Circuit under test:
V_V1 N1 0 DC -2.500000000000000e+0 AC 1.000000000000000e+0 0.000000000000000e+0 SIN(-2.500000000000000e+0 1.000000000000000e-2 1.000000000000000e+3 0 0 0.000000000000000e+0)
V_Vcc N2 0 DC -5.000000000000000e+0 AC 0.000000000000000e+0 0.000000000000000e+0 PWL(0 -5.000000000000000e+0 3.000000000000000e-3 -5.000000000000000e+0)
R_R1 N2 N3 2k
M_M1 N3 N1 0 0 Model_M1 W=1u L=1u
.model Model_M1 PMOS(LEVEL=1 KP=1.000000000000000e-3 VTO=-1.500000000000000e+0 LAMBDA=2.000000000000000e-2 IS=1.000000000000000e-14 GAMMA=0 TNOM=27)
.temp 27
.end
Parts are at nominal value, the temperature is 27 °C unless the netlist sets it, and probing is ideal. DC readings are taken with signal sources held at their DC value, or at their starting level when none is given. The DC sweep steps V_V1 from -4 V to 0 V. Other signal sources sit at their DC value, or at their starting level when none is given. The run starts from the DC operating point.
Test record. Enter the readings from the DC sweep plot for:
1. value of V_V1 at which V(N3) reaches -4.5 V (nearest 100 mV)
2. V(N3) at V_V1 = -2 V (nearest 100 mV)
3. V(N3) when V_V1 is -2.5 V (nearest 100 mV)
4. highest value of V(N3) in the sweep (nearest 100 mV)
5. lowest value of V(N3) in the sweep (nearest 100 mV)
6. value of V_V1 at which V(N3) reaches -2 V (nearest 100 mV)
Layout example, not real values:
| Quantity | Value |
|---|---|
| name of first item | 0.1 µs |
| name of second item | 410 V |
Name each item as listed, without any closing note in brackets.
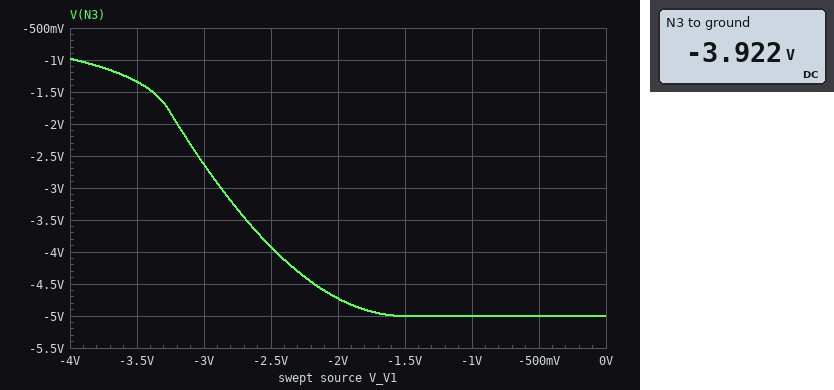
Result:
| Quantity | Value |
|---|---|
| value of V_V1 at which V(N3) reaches -4.5 V | -2.2 V |
| V(N3) at V_V1 = -2 V | -4.7 V |
| V(N3) when V_V1 is -2.5 V | -3.9 V |
| highest value of V(N3) in the sweep | -1.0 V |
| lowest value of V(N3) in the sweep | -5.0 V |
| value of V_V1 at which V(N3) reaches -2 V | -3.2 V |
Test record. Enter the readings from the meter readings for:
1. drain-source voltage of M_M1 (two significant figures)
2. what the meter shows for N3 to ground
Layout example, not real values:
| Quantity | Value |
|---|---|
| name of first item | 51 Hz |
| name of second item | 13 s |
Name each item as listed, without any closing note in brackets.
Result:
| Quantity | Value |
|---|---|
| drain-source voltage of M_M1 | -3.9 V |
| what the meter shows for N3 to ground | -3.922 V |
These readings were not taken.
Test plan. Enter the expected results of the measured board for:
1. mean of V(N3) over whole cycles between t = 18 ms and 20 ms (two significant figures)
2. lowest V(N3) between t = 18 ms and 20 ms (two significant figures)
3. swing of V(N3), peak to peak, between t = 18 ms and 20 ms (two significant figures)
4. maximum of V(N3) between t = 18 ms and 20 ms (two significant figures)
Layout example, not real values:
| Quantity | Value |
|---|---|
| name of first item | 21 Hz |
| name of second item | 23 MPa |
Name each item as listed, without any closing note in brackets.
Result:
| Quantity | Value |
|---|---|
| mean of V(N3) over whole cycles between t = 18 ms and 20 ms | -3.9 V |
| lowest V(N3) between t = 18 ms and 20 ms | -3.9 V |
| swing of V(N3), peak to peak, between t = 18 ms and 20 ms | 42 mV |
| maximum of V(N3) between t = 18 ms and 20 ms | -3.9 V |
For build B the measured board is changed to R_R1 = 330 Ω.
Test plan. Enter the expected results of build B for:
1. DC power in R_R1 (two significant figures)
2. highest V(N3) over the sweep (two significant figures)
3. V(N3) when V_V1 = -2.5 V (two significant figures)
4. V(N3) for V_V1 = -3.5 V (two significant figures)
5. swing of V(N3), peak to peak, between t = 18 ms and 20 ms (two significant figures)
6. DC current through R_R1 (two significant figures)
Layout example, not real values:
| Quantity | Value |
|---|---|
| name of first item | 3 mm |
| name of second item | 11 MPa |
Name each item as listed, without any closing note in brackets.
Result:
| Quantity | Value |
|---|---|
| DC power in R_R1 | 99 µW |
| highest V(N3) over the sweep | -3.9 V |
| V(N3) when V_V1 = -2.5 V | -4.8 V |
| V(N3) for V_V1 = -3.5 V | -4.3 V |
| swing of V(N3), peak to peak, between t = 18 ms and 20 ms | 7.2 mV |
| DC current through R_R1 | 550 µA |
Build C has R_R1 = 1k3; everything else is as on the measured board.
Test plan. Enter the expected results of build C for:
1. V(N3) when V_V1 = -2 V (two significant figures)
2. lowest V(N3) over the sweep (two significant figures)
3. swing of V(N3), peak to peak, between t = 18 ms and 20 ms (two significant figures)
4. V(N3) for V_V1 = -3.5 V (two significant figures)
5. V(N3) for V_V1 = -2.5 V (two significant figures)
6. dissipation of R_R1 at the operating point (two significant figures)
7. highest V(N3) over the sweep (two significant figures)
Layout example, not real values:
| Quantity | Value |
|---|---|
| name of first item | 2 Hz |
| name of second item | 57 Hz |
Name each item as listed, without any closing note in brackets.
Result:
| Quantity | Value |
|---|---|
| V(N3) when V_V1 = -2 V | -4.8 V |
| lowest V(N3) over the sweep | -5.0 V |
| swing of V(N3), peak to peak, between t = 18 ms and 20 ms | 28 mV |
| V(N3) for V_V1 = -3.5 V | -2.3 V |
| V(N3) for V_V1 = -2.5 V | -4.3 V |
| dissipation of R_R1 at the operating point | 380 µW |
| highest V(N3) over the sweep | -1.5 V |
